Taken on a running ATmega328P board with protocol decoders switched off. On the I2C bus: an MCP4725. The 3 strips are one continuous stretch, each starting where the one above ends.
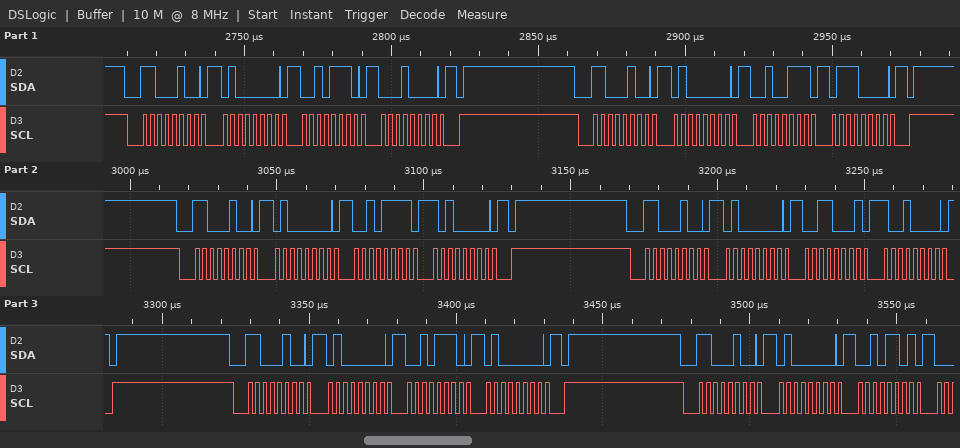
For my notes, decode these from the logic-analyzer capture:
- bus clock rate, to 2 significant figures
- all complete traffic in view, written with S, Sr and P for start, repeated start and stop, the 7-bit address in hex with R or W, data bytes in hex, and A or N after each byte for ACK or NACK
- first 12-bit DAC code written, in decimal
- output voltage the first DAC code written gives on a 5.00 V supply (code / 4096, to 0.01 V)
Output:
400 kHz
S 62W A 40 A 2E A 10 A P S 62W A 40 A 27 A 70 A P S 62W A 40 A 2F A A0 A P S 62W A 40 A 31 A 90 A P S 62W A 40 A 2E A 40 A P S 62W A 40 A 2D A
737
0.90 V
